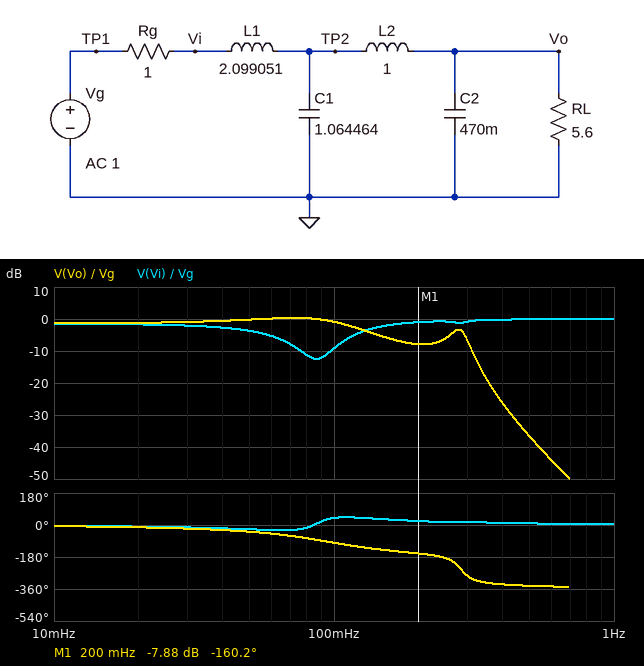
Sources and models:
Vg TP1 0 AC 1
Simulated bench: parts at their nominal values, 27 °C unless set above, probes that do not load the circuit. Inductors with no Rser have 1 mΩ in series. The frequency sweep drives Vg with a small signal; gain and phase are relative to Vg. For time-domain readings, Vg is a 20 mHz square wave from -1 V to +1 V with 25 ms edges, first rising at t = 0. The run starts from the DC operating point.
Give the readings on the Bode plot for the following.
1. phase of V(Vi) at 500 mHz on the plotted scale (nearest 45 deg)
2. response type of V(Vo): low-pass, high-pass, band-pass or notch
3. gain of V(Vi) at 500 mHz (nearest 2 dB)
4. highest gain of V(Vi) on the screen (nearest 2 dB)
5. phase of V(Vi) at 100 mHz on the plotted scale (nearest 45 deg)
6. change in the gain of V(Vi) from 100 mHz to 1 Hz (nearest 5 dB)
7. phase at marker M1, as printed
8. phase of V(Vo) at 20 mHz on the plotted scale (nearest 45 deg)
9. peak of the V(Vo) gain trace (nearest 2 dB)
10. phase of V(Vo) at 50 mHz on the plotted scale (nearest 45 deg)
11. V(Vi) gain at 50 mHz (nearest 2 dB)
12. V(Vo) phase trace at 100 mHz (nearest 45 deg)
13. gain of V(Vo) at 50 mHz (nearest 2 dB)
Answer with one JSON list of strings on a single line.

["0 deg", "low-pass", "0 dB", "0 dB", "45 deg", "10 dB", "-160.2 deg", "0 deg", "0 dB", "-45 deg", "-4 dB", "-90 deg", "0 dB"]
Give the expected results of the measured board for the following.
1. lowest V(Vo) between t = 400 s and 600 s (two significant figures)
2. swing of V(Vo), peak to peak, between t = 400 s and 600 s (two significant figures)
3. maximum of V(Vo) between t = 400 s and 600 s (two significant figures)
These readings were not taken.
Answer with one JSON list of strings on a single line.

["-1.2 V", "2.4 V", "1.2 V"]
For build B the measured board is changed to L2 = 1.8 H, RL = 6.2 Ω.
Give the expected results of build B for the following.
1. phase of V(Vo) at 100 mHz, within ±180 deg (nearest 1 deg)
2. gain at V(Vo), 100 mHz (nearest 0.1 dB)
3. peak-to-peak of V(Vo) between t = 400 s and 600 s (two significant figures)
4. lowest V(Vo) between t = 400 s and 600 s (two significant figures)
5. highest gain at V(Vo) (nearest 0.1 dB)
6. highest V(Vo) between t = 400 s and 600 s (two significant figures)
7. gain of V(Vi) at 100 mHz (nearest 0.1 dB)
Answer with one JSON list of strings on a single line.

["-106 deg", "-0.1 dB", "2.6 V", "-1.3 V", "0.9 dB", "1.3 V", "-8.3 dB"]
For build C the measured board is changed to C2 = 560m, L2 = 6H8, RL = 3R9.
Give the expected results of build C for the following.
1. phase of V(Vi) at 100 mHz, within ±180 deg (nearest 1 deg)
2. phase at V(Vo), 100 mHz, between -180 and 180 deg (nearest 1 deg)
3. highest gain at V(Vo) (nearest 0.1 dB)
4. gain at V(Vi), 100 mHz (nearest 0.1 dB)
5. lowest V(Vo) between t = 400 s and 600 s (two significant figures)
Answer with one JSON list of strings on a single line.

["-16 deg", "-154 deg", "-0.5 dB", "-4.0 dB", "-1.2 V"]
